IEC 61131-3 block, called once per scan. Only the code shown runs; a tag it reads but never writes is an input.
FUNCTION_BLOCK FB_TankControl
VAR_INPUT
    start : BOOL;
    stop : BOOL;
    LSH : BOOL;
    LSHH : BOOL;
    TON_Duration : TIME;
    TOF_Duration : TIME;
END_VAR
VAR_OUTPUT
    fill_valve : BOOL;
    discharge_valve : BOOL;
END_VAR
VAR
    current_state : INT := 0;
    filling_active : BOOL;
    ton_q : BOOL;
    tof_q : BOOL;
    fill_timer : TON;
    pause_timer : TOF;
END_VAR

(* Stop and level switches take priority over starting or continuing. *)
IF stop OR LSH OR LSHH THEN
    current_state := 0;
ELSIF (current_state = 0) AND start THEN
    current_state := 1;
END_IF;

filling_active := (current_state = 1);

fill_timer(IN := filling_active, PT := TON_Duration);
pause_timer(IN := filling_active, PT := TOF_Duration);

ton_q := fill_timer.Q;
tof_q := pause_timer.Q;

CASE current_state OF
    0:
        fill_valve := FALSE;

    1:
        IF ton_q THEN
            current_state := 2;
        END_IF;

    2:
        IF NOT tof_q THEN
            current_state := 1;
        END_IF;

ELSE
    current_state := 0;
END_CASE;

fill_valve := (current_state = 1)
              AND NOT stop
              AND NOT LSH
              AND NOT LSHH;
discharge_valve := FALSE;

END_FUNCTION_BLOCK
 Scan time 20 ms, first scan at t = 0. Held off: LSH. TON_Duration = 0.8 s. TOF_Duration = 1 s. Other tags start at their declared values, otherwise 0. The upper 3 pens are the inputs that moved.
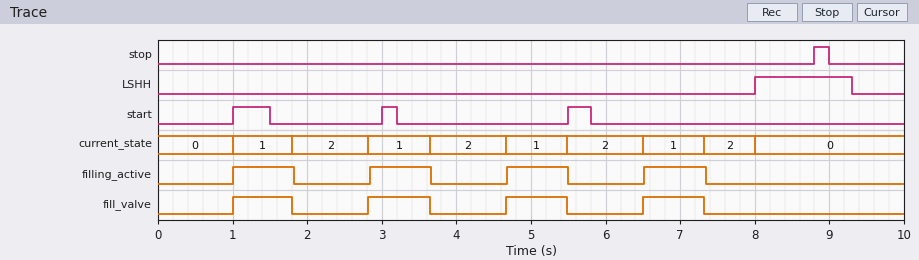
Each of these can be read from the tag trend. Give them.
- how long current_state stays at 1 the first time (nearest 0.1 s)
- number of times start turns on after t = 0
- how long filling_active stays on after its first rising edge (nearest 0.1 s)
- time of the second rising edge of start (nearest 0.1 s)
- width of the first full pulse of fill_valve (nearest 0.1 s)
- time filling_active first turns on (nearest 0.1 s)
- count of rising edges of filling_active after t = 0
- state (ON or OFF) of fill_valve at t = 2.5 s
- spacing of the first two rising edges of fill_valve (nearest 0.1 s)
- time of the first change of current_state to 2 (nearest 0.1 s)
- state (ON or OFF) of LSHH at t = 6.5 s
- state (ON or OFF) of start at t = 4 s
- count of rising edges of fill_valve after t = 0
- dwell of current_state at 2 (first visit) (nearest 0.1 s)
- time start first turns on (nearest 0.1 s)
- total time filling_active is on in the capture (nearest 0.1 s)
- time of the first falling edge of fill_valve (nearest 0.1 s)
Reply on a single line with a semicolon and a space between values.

0.8 s; 3; 0.8 s; 3.0 s; 0.8 s; 1.0 s; 4; OFF; 1.8 s; 1.8 s; OFF; OFF; 4; 1.0 s; 1.0 s; 3.3 s; 1.8 s
